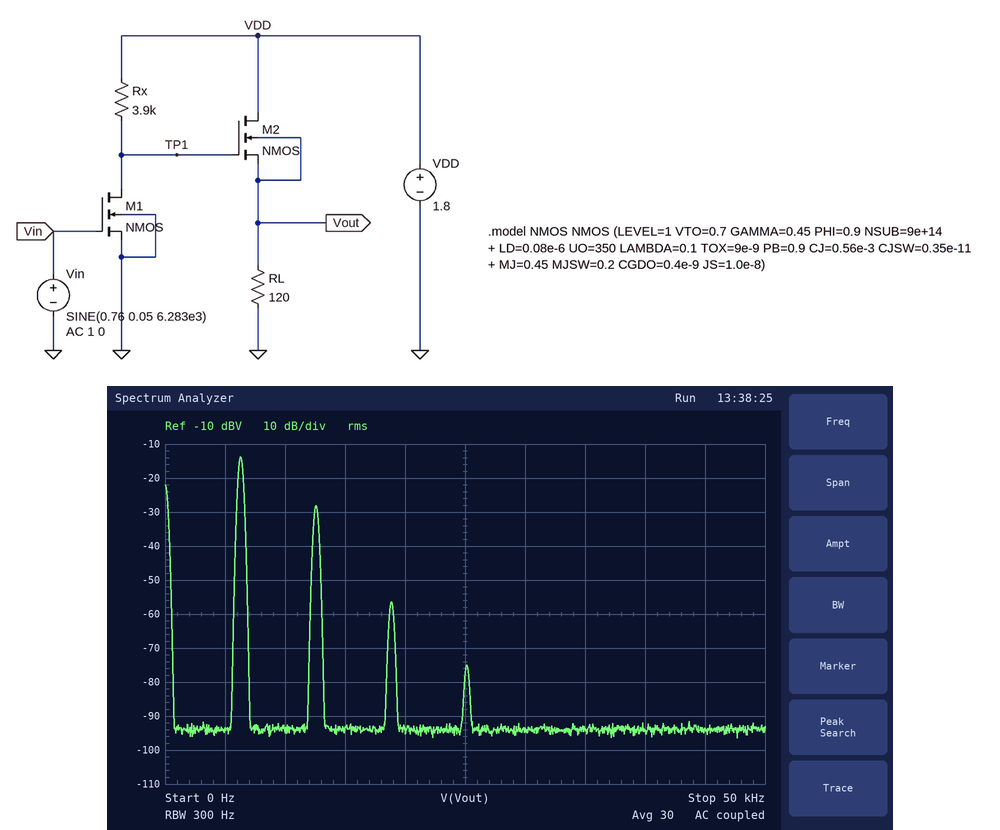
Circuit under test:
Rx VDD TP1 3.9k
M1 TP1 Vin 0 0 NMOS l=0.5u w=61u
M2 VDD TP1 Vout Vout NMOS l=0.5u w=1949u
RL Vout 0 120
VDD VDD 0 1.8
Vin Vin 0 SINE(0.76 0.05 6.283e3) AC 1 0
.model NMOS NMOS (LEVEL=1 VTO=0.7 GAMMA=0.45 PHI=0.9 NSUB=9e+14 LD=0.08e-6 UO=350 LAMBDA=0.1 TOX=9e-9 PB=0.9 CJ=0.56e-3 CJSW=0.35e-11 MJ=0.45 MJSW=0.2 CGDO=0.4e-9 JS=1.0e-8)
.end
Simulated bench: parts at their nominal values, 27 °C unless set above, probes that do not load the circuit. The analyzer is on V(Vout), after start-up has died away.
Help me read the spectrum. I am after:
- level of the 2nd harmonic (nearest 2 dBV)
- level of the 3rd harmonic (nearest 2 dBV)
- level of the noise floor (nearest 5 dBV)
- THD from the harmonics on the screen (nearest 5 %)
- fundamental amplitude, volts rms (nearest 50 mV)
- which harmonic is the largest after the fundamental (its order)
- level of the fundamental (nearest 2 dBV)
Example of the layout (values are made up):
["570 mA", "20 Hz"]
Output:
["-28 dBV", "-56 dBV", "-95 dBV", "20 %", "200 mV", "2", "-14 dBV"]
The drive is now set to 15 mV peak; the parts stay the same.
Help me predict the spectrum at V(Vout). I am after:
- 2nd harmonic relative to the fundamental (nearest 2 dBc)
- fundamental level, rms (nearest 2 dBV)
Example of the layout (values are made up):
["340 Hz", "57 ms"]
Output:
["-24 dBc", "-24 dBV"]
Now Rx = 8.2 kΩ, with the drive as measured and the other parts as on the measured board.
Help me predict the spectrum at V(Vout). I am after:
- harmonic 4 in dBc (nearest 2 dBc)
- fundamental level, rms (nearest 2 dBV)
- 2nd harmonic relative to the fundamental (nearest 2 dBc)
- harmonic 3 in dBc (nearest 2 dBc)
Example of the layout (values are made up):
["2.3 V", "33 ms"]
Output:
["-28 dBc", "-8 dBV", "-18 dBc", "-22 dBc"]
